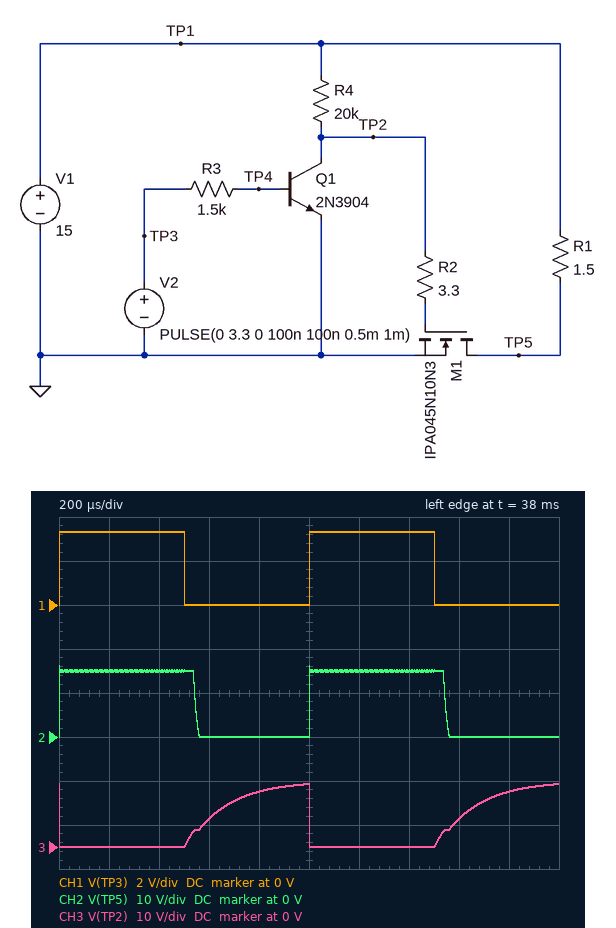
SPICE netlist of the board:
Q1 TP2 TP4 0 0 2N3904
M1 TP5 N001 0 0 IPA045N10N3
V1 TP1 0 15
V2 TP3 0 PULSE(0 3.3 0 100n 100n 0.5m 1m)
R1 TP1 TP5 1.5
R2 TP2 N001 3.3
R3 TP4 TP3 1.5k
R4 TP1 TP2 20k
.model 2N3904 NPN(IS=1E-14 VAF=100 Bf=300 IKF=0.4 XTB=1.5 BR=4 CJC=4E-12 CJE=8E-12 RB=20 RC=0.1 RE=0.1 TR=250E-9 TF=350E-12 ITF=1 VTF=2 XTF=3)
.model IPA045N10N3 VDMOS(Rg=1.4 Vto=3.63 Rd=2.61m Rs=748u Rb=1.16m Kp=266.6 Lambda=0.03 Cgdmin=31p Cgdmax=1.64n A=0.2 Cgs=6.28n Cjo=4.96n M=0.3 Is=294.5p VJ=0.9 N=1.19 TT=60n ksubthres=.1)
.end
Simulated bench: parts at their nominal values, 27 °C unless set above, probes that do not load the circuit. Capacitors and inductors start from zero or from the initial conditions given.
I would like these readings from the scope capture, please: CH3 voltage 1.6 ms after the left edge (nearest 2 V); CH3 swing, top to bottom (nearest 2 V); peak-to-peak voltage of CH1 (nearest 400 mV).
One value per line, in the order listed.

6 V
14 V
3.2 V
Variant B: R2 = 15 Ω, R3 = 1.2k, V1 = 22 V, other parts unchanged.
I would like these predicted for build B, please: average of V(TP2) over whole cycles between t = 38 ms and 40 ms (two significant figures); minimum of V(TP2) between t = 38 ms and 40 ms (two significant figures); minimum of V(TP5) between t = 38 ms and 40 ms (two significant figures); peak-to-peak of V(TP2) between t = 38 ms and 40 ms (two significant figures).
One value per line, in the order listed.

7.5 V
2.4 mV
52 mV
21 V
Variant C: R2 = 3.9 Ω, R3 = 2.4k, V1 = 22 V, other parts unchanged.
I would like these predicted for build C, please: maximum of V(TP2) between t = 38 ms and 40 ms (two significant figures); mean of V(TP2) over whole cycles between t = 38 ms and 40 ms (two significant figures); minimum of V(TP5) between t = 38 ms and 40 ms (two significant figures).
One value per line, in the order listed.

21 V
7.5 V
52 mV
